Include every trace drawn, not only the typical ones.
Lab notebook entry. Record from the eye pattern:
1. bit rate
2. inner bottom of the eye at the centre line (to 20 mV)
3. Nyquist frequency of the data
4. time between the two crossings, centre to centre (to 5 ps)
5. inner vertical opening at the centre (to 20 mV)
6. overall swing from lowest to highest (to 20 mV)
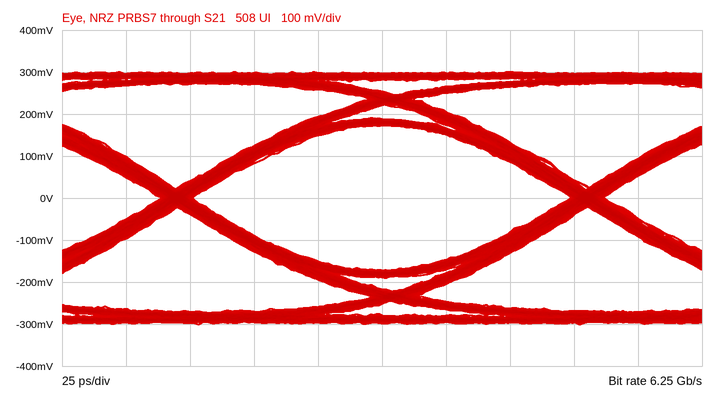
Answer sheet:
6.25 Gb/s
-180 mV
3.125 GHz
160 ps
340 mV
600 mV
